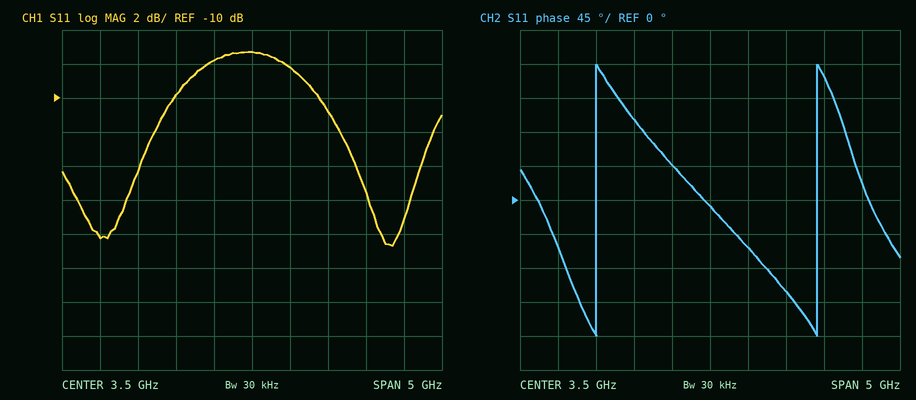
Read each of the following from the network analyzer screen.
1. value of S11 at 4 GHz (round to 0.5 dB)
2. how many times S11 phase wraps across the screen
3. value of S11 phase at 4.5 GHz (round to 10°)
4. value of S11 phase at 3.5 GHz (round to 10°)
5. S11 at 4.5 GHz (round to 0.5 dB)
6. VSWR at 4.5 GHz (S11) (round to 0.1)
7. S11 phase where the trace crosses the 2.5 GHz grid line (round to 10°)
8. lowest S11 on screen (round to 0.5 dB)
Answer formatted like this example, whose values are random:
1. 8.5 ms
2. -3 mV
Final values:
1. -8.0 dB
2. 2
3. -120°
4. -10°
5. -11.0 dB
6. 1.8
7. 110°
8. -18.5 dB
